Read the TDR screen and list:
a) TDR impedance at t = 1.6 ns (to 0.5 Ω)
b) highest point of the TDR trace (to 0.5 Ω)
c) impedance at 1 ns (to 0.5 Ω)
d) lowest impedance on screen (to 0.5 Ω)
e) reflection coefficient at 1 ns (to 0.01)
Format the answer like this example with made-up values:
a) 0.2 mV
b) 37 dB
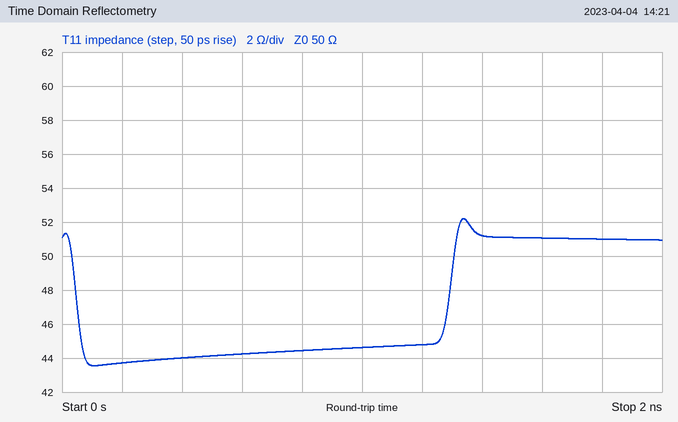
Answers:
a) 51.0 Ω
b) 52.0 Ω
c) 44.5 Ω
d) 43.5 Ω
e) -0.06
